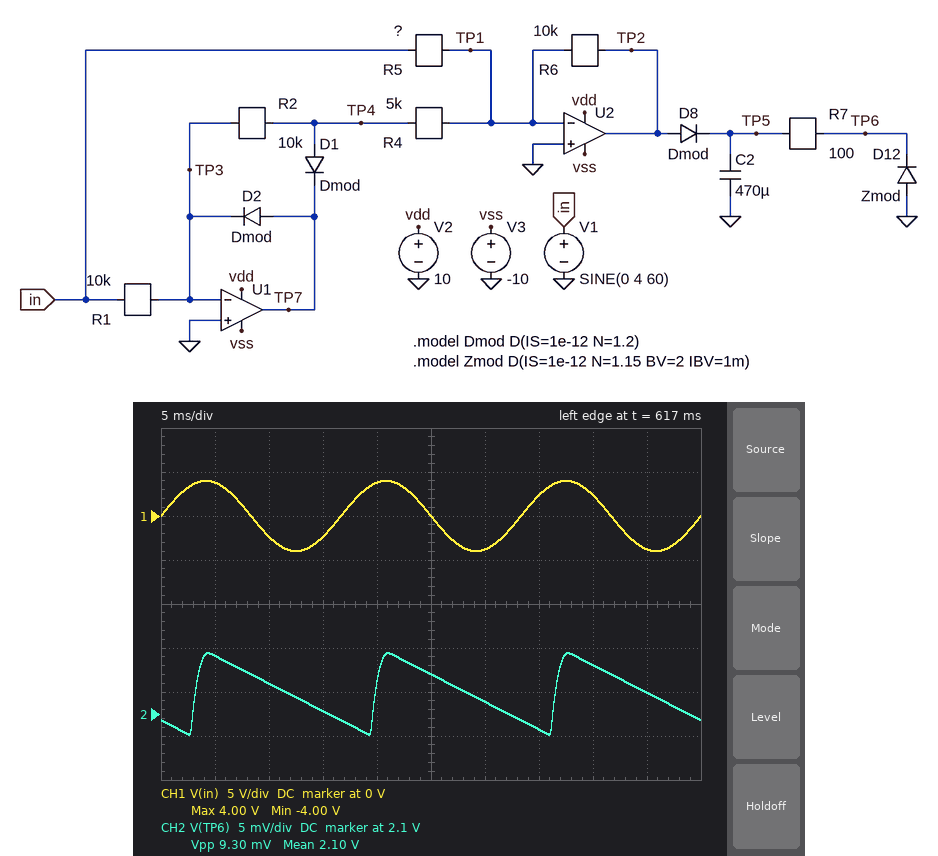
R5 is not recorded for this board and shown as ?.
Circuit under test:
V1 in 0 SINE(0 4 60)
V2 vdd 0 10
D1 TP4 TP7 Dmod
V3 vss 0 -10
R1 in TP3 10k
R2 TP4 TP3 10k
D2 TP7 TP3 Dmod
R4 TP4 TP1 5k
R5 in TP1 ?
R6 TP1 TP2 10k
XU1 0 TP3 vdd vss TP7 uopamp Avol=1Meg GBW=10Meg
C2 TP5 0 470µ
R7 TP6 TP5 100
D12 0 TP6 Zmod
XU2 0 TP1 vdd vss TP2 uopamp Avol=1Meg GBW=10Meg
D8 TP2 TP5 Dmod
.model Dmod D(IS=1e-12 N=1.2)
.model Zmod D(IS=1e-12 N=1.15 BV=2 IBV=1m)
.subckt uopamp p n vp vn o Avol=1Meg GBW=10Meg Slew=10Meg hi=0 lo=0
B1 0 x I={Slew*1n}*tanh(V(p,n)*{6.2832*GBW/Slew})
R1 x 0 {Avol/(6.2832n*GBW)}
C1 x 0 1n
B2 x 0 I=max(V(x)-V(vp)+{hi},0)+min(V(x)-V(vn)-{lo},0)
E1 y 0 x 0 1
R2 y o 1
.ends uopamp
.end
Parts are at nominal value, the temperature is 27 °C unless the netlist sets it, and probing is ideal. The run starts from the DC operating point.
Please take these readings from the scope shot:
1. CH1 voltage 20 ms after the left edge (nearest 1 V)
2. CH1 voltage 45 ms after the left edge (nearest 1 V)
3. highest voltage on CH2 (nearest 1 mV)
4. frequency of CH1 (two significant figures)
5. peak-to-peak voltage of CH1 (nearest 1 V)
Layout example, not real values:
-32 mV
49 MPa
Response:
4 V
-4 V
2.107 V
60 Hz
8 V
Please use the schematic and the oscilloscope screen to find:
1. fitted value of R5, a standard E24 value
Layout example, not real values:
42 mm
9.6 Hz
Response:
27 kΩ
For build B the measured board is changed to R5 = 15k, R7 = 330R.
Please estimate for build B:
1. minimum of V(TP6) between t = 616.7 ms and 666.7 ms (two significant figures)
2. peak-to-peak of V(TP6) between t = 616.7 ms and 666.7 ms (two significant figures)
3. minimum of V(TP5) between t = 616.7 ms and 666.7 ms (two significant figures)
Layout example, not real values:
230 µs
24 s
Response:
2.1 V
2.9 mV
4.3 V
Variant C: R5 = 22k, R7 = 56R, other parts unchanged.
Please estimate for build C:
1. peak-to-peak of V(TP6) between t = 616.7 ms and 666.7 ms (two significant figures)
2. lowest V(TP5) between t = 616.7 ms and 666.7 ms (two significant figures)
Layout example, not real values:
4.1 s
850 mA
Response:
16 mV
4.0 V
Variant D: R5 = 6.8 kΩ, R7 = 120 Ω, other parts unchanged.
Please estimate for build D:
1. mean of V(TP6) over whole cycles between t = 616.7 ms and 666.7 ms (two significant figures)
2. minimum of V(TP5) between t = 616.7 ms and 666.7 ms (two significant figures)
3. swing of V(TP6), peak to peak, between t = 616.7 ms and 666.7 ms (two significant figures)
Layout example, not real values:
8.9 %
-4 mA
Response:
2.1 V
4.4 V
7.8 mV
